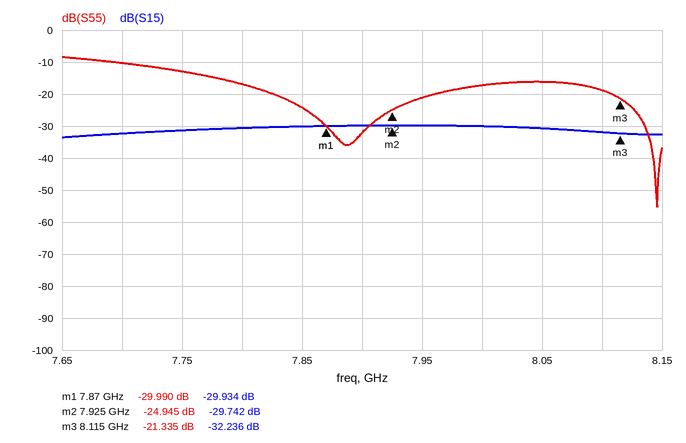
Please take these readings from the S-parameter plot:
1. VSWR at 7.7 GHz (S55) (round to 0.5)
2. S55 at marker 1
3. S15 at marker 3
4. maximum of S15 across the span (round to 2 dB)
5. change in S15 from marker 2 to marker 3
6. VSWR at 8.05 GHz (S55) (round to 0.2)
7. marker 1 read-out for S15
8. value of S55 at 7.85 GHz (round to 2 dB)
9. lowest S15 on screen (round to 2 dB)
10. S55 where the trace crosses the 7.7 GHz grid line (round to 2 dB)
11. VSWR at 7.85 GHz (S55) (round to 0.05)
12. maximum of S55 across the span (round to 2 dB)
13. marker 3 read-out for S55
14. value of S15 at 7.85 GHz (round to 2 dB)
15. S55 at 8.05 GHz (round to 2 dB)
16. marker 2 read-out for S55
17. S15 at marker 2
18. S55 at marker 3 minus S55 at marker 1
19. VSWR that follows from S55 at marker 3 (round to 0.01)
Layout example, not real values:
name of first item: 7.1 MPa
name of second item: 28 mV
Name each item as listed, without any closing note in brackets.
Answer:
VSWR at 7.7 GHz (S55): 2.0
S55 at marker 1: -29.990 dB
S15 at marker 3: -32.236 dB
maximum of S15 across the span: -30 dB
change in S15 from marker 2 to marker 3: -2.494 dB
VSWR at 8.05 GHz (S55): 1.4
marker 1 read-out for S15: -29.934 dB
value of S55 at 7.85 GHz: -24 dB
lowest S15 on screen: -34 dB
S55 where the trace crosses the 7.7 GHz grid line: -10 dB
VSWR at 7.85 GHz (S55): 1.15
maximum of S55 across the span: -8 dB
marker 3 read-out for S55: -21.335 dB
value of S15 at 7.85 GHz: -30 dB
S55 at 8.05 GHz: -16 dB
marker 2 read-out for S55: -24.945 dB
S15 at marker 2: -29.742 dB
S55 at marker 3 minus S55 at marker 1: 8.655 dB
VSWR that follows from S55 at marker 3: 1.19
